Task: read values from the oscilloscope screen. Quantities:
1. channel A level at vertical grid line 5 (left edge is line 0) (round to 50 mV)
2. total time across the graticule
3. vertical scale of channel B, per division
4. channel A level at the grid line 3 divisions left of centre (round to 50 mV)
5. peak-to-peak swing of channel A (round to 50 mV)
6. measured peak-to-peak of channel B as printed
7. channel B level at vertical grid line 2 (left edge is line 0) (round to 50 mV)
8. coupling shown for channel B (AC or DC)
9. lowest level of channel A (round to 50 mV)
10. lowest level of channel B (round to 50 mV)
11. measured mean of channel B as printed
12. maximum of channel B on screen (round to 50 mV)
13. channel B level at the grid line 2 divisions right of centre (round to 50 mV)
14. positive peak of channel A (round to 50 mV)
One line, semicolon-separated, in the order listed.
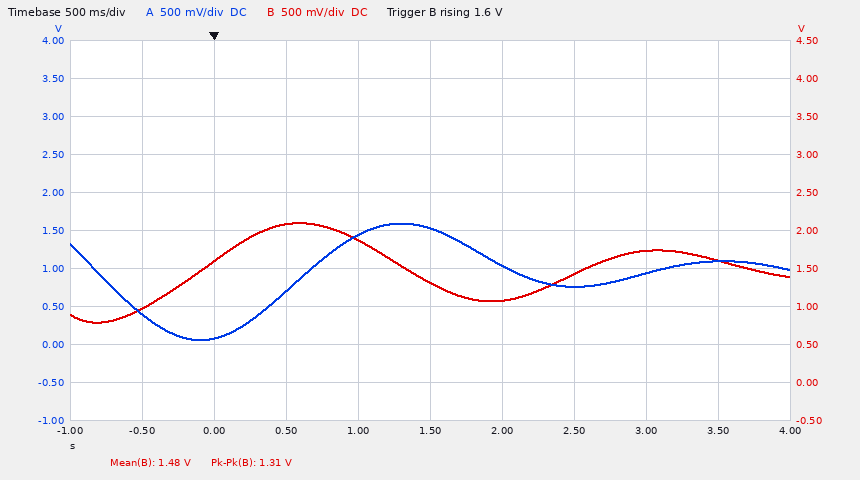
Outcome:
1.55 V; 5 s; 500 mV; 100 mV; 1.55 V; 1.31 V; 1.60 V; DC; 50 mV; 800 mV; 1.48 V; 2.10 V; 1.45 V; 1.60 V
